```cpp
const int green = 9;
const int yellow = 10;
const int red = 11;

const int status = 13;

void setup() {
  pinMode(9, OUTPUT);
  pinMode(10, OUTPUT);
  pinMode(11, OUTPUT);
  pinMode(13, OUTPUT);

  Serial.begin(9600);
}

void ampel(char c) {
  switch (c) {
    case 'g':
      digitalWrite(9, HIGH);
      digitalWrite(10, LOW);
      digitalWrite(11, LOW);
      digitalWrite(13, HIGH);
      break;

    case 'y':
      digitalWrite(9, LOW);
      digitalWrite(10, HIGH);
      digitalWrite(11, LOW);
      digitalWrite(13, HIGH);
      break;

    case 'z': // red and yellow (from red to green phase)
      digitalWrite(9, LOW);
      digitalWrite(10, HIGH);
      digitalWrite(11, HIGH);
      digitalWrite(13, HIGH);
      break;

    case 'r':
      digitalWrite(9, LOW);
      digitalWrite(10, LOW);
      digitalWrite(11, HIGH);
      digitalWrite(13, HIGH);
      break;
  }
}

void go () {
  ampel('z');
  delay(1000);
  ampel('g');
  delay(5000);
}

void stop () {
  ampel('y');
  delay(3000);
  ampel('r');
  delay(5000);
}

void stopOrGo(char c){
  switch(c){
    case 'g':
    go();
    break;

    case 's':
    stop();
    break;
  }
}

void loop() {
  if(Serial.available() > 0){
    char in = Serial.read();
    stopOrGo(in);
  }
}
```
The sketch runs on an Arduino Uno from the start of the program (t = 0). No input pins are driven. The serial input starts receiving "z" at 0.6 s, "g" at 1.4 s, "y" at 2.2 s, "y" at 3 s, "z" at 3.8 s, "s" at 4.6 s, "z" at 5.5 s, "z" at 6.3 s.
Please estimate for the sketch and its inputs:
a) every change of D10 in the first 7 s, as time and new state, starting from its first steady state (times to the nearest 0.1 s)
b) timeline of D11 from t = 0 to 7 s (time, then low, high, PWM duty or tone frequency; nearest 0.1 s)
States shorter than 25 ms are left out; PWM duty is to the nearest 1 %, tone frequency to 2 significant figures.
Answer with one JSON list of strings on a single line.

["0 s low; 1.4 s high; 2.4 s low", "0 s low; 1.4 s high; 2.4 s low"]
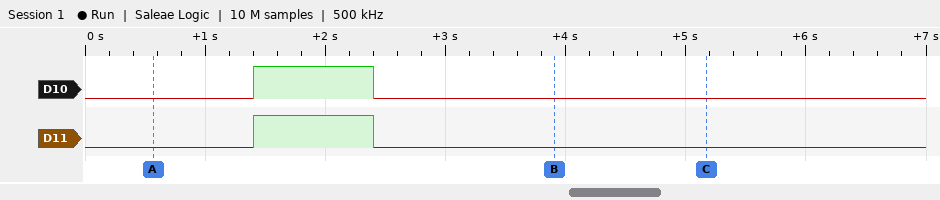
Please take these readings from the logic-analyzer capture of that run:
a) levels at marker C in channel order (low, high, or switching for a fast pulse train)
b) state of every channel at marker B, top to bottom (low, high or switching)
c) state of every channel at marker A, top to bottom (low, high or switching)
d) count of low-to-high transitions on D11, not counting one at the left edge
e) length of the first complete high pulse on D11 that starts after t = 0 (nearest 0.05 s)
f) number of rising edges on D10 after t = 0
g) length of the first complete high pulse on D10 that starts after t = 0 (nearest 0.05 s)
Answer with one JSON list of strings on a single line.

["D10 low, D11 low", "D10 low, D11 low", "D10 low, D11 low", "1", "1.00 s", "1", "1.00 s"]
